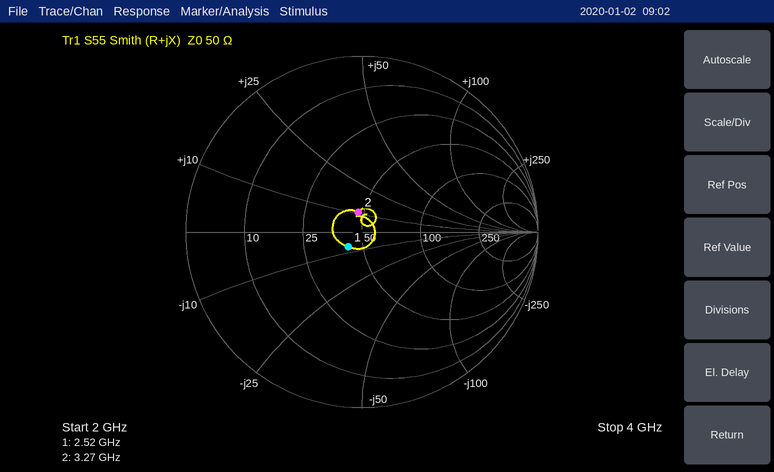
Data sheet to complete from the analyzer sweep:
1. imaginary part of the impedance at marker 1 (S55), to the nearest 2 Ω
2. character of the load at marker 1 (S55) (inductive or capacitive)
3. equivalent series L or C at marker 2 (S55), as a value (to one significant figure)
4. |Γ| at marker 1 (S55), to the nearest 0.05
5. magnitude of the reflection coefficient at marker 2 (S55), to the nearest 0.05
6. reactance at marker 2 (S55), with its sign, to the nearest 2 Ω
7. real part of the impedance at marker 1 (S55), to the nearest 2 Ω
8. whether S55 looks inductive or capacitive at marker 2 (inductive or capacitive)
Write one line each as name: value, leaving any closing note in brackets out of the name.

imaginary part of the impedance at marker 1 (S55), to the nearest 2 Ω: -8 Ω
character of the load at marker 1 (S55): capacitive
equivalent series L or C at marker 2 (S55), as a value: 500 pH
|Γ| at marker 1 (S55), to the nearest 0.05: 0.10
magnitude of the reflection coefficient at marker 2 (S55), to the nearest 0.05: 0.10
reactance at marker 2 (S55), with its sign, to the nearest 2 Ω: +10 Ω
real part of the impedance at marker 1 (S55), to the nearest 2 Ω: 42 Ω
whether S55 looks inductive or capacitive at marker 2: inductive
